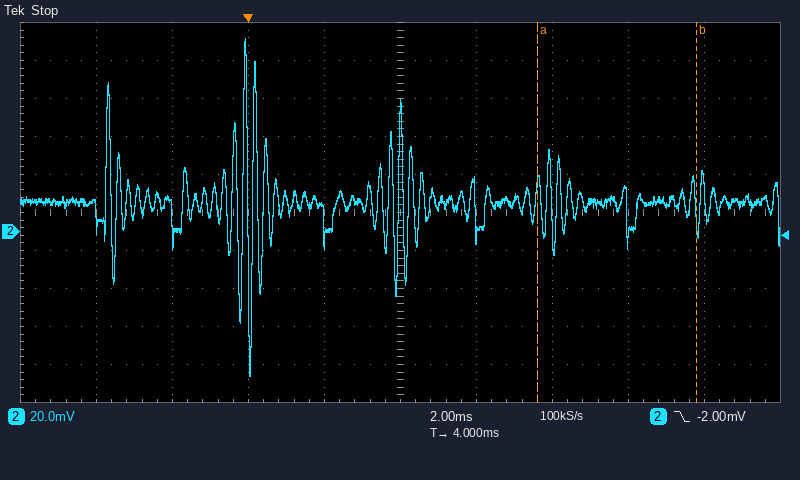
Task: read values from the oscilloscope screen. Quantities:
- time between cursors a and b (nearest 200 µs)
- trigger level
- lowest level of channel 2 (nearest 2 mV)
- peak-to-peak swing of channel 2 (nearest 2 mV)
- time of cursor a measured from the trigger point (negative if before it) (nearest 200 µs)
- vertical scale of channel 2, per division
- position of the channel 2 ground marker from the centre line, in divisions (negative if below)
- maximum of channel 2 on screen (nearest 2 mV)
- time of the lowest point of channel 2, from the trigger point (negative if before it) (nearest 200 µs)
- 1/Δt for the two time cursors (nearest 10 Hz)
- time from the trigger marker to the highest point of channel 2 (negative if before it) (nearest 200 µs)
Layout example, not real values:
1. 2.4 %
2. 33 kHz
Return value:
1. 4.2 ms
2. -2.00 mV
3. -76 mV
4. 178 mV
5. +7.6 ms
6. 20 mV
7. -0.5 div
8. 102 mV
9. 0.0 ms
10. 240 Hz
11. 0.0 ms
